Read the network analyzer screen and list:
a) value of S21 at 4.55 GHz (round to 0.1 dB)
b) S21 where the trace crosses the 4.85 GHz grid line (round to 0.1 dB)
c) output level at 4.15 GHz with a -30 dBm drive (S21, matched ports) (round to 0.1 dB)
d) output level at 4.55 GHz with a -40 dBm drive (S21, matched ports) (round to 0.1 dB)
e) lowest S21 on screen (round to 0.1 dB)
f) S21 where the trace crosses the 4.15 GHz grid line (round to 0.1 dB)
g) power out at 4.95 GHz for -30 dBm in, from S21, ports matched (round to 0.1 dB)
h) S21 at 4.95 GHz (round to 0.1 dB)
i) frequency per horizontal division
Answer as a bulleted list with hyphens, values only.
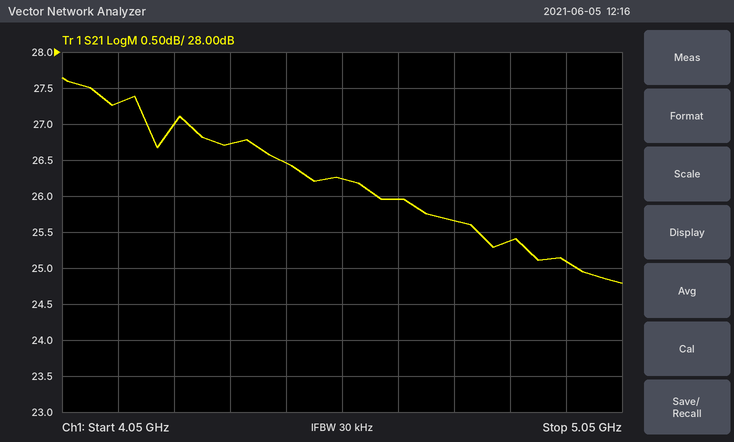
- 26.2 dB
- 25.4 dB
- -2.7 dBm
- -13.8 dBm
- 24.8 dB
- 27.3 dB
- -4.9 dBm
- 25.1 dB
- 100 MHz
